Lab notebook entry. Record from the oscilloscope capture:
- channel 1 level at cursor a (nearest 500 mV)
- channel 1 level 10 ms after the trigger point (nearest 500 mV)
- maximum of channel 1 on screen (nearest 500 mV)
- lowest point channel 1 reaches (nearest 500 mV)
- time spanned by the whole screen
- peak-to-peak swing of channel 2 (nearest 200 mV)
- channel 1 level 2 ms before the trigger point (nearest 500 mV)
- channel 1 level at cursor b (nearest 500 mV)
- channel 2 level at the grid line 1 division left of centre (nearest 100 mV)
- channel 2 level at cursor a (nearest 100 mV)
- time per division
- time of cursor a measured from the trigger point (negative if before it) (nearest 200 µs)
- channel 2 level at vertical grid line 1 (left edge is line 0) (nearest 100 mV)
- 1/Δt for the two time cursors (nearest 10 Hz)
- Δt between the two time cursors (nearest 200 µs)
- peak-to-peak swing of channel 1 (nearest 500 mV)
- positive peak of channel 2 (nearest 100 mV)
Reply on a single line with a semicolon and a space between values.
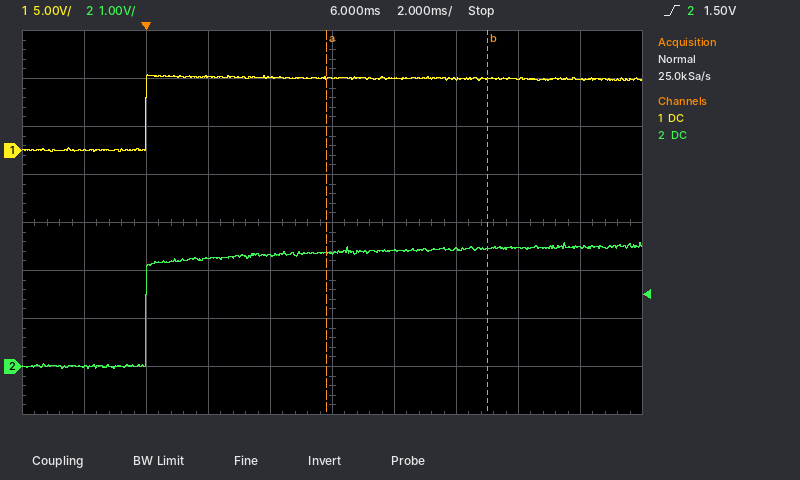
7.5 V; 7.5 V; 8.0 V; 0.0 V; 20 ms; 2.6 V; 0.0 V; 7.5 V; 2.3 V; 2.4 V; 2 ms; +5.8 ms; 0.0 V; 190 Hz; 5.2 ms; 8.0 V; 2.6 V
